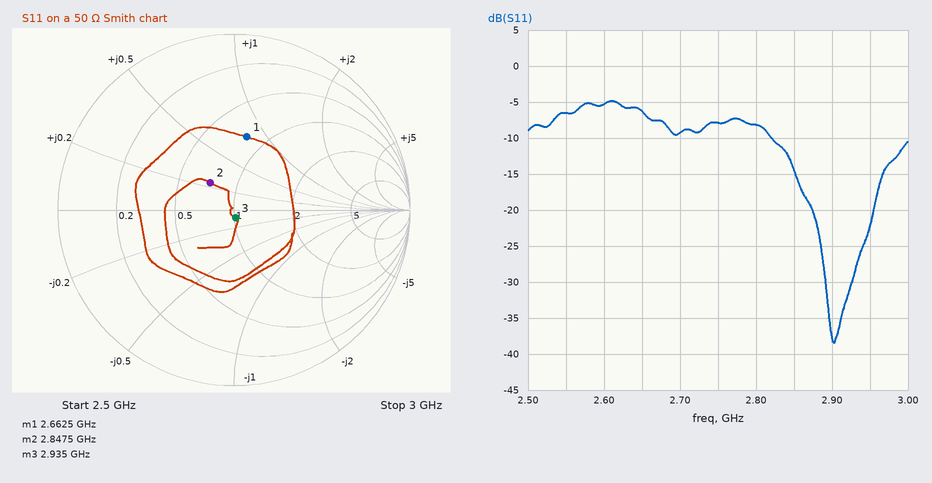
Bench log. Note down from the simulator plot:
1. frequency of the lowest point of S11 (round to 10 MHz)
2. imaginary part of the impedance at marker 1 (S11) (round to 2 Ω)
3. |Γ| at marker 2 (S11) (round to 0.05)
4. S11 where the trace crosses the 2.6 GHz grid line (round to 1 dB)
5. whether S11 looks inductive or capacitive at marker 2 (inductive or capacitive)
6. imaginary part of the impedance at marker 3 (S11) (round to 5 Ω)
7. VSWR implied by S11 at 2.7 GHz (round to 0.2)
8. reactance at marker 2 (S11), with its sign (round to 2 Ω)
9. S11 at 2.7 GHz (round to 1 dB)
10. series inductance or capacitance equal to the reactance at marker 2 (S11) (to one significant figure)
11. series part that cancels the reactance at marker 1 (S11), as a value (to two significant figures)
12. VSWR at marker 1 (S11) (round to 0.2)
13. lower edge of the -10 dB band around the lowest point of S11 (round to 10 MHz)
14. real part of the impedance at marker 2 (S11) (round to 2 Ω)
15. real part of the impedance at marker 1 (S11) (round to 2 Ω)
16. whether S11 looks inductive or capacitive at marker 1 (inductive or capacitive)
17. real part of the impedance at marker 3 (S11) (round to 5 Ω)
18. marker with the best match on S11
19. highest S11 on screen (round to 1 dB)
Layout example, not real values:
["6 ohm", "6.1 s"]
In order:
["2.90 GHz", "+40 Ω", "0.20", "-5 dB", "inductive", "-5 Ω", "2.0", "+12 Ω", "-9 dB", "700 pH", "1.5 pF", "2.4", "2.82 GHz", "36 Ω", "40 Ω", "inductive", "50 Ω", "marker 3", "-5 dB"]
